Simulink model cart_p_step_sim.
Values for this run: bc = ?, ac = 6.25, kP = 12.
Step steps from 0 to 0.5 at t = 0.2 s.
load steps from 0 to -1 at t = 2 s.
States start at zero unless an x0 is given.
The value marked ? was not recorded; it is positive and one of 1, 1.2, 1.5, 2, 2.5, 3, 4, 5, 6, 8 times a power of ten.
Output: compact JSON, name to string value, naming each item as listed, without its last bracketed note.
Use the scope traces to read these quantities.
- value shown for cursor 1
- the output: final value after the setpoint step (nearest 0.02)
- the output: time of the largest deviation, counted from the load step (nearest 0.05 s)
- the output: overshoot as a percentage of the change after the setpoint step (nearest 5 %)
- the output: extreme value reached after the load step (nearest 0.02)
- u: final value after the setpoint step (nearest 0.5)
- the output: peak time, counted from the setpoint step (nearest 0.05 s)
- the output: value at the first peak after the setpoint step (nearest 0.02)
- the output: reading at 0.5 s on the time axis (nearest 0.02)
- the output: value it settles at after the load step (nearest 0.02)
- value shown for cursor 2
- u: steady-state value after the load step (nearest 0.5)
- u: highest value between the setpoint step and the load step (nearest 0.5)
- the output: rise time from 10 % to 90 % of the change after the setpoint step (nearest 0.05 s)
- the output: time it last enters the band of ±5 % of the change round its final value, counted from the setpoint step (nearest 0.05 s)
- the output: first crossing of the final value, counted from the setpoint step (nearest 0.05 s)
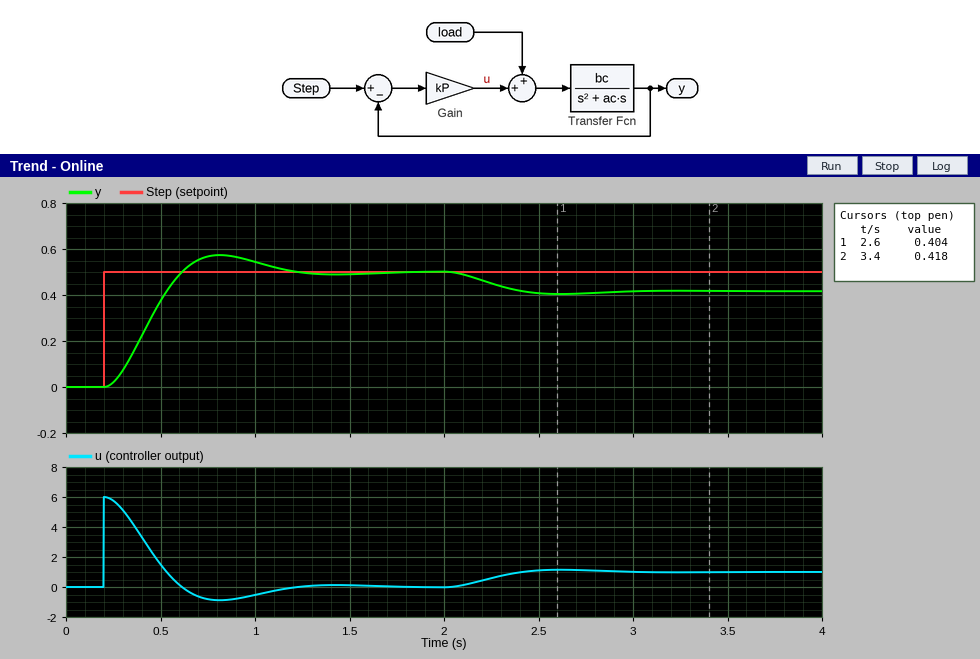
{"value shown for cursor 1": "0.404", "the output: final value after the setpoint step": "0.50", "the output: time of the largest deviation, counted from the load step": "0.60 s", "the output: overshoot as a percentage of the change after the setpoint step": "15 %", "the output: extreme value reached after the load step": "0.40", "u: final value after the setpoint step": "0.0", "the output: peak time, counted from the setpoint step": "0.60 s", "the output: value at the first peak after the setpoint step": "0.58", "the output: reading at 0.5 s on the time axis": "0.38", "the output: value it settles at after the load step": "0.42", "value shown for cursor 2": "0.418", "u: steady-state value after the load step": "1.0", "u: highest value between the setpoint step and the load step": "6.0", "the output: rise time from 10 % to 90 % of the change after the setpoint step": "0.30 s", "the output: time it last enters the band of ±5 % of the change round its final value, counted from the setpoint step": "0.90 s", "the output: first crossing of the final value, counted from the setpoint step": "0.40 s"}
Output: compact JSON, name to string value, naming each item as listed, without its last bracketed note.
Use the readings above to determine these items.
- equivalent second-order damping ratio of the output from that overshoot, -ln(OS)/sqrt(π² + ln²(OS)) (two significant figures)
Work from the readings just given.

{"equivalent second-order damping ratio of the output from that overshoot, -ln(OS)/sqrt(π² + ln²(OS))": "0.52"}
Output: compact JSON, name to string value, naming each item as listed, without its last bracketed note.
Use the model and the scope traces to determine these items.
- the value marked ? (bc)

{"the value marked ?": "3"}
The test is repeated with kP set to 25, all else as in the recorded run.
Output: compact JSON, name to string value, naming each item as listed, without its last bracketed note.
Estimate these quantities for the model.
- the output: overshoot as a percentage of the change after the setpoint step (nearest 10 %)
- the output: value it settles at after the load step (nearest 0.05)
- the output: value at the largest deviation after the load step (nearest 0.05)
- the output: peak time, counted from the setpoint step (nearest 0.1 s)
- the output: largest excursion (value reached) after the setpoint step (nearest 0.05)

{"the output: overshoot as a percentage of the change after the setpoint step": "30 %", "the output: value it settles at after the load step": "0.45", "the output: value at the largest deviation after the load step": "0.45", "the output: peak time, counted from the setpoint step": "0.4 s", "the output: largest excursion (value reached) after the setpoint step": "0.65"}
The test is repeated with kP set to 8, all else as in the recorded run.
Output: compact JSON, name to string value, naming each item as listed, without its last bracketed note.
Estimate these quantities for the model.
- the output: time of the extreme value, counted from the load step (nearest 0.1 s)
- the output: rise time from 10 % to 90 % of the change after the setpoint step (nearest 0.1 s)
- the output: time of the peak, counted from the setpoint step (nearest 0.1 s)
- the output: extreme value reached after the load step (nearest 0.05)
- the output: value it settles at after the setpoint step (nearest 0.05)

{"the output: time of the extreme value, counted from the load step": "0.8 s", "the output: rise time from 10 % to 90 % of the change after the setpoint step": "0.4 s", "the output: time of the peak, counted from the setpoint step": "0.8 s", "the output: extreme value reached after the load step": "0.35", "the output: value it settles at after the setpoint step": "0.50"}
